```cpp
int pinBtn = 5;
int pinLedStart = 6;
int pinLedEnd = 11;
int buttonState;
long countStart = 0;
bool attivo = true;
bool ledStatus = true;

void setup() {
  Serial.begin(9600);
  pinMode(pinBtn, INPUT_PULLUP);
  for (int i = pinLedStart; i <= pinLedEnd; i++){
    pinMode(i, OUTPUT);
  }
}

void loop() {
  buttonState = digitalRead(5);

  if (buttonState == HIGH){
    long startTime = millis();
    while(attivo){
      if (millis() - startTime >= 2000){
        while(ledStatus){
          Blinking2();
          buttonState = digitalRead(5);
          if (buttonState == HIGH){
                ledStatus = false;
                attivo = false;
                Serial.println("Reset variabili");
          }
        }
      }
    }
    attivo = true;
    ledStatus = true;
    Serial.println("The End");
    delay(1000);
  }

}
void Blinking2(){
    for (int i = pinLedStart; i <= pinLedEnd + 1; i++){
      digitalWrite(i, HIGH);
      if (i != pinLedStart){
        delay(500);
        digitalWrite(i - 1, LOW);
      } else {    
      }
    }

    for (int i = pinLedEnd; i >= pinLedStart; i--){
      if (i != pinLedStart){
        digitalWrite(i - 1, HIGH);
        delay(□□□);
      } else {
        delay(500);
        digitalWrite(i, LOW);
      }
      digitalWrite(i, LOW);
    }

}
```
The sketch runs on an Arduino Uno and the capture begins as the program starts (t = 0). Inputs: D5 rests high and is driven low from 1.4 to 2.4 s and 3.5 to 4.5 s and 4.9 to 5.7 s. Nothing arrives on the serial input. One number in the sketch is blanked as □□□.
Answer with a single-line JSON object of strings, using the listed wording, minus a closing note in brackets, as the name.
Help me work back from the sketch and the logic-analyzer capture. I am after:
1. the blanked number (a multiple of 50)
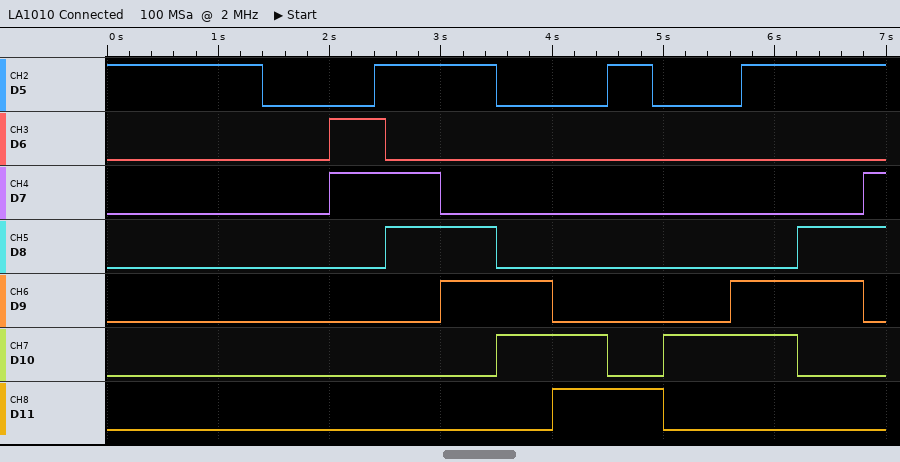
{"the blanked number": "600"}
